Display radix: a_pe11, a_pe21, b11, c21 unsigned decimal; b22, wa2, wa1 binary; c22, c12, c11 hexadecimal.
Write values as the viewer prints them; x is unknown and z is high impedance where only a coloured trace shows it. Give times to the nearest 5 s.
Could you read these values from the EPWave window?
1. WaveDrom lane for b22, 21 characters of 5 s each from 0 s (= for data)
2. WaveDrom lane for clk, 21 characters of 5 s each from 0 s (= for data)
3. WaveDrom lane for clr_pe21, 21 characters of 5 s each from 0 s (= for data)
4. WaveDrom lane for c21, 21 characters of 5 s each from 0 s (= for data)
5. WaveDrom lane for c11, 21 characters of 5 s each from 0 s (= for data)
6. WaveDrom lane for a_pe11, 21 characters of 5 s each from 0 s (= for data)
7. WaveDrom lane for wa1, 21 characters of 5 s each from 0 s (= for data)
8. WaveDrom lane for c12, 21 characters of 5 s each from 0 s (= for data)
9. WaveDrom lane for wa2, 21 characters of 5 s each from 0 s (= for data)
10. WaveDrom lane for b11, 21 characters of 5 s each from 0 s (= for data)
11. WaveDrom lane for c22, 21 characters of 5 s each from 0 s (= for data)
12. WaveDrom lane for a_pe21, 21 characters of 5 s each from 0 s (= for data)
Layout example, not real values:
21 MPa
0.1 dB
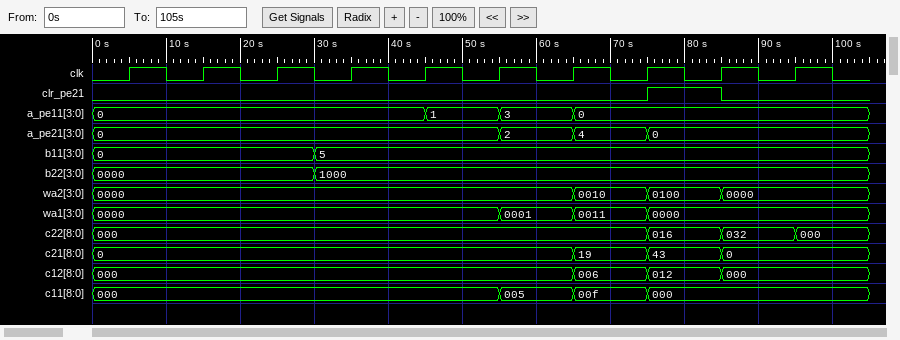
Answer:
{name: 'b22', wave: '=.....=..............', data: '0000 1000'}
{name: 'clk', wave: '010101010101010101010'}
{name: 'clr_pe21', wave: '0..............1.0...'}
{name: 'c21', wave: '=............=.=.=...', data: '0 19 43 0'}
{name: 'c11', wave: '=..........=.=.=.....', data: '000 005 00f 000'}
{name: 'a_pe11', wave: '=........=.=.=.......', data: '0 1 3 0'}
{name: 'wa1', wave: '=..........=.=.=.....', data: '0000 0001 0011 0000'}
{name: 'c12', wave: '=............=.=.=...', data: '000 006 012 000'}
{name: 'wa2', wave: '=............=.=.=...', data: '0000 0010 0100 0000'}
{name: 'b11', wave: '=.....=..............', data: '0 5'}
{name: 'c22', wave: '=..............=.=.=.', data: '000 016 032 000'}
{name: 'a_pe21', wave: '=..........=.=.=.....', data: '0 2 4 0'}
